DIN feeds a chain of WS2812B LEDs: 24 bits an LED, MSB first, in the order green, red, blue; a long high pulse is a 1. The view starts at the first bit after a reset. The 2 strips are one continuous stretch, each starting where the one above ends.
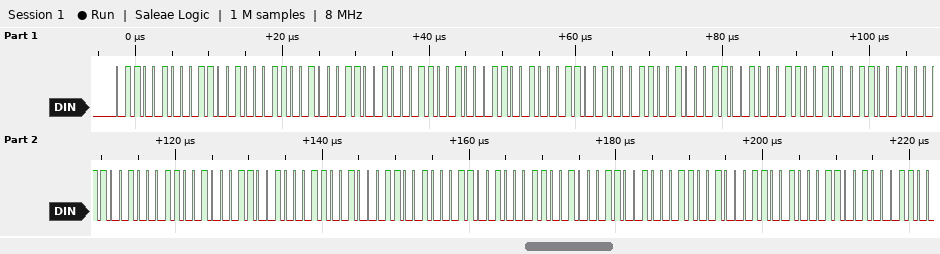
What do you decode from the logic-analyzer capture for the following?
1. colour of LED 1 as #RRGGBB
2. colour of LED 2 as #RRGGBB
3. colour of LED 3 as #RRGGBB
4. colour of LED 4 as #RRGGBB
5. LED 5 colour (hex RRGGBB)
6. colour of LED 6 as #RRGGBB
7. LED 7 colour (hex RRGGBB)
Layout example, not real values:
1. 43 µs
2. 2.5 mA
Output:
1. #646464
2. #646464
3. #646464
4. #646464
5. #646464
6. #646464
7. #646464
